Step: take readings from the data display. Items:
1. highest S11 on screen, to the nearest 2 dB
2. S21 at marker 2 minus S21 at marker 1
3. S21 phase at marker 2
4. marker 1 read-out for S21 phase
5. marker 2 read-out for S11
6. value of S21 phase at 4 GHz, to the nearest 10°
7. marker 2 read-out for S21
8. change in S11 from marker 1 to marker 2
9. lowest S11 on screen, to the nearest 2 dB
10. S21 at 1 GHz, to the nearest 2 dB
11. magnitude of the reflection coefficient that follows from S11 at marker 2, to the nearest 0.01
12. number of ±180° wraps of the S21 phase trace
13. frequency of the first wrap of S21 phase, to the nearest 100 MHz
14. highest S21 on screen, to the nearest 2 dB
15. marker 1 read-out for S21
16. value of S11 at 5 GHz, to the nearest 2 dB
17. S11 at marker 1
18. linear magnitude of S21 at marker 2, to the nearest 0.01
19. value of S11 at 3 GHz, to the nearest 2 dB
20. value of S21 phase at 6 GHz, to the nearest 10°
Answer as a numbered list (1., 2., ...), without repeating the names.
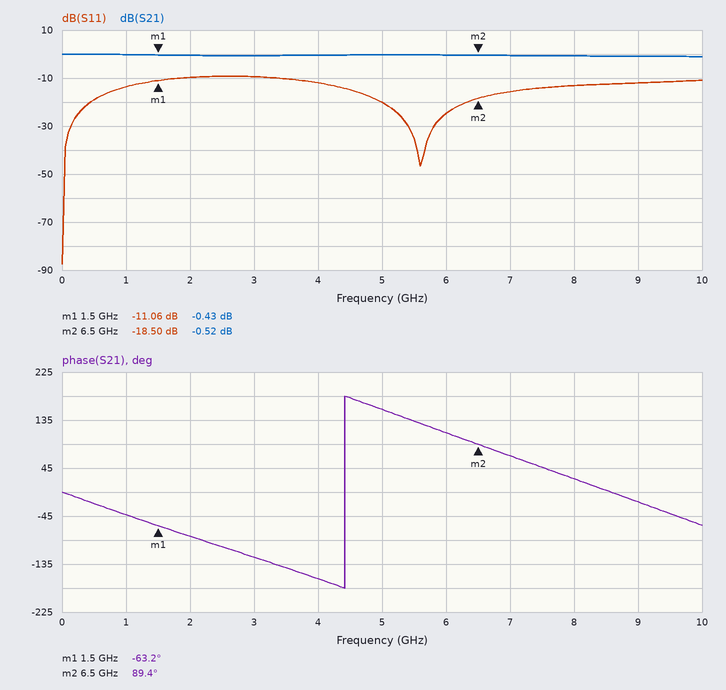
1. -10 dB
2. -0.09 dB
3. 89.4°
4. -63.2°
5. -18.50 dB
6. -160°
7. -0.52 dB
8. -7.44 dB
9. -88 dB
10. 0 dB
11. 0.12
12. 1
13. 4.4 GHz
14. 0 dB
15. -0.43 dB
16. -20 dB
17. -11.06 dB
18. 0.94
19. -10 dB
20. 110°
